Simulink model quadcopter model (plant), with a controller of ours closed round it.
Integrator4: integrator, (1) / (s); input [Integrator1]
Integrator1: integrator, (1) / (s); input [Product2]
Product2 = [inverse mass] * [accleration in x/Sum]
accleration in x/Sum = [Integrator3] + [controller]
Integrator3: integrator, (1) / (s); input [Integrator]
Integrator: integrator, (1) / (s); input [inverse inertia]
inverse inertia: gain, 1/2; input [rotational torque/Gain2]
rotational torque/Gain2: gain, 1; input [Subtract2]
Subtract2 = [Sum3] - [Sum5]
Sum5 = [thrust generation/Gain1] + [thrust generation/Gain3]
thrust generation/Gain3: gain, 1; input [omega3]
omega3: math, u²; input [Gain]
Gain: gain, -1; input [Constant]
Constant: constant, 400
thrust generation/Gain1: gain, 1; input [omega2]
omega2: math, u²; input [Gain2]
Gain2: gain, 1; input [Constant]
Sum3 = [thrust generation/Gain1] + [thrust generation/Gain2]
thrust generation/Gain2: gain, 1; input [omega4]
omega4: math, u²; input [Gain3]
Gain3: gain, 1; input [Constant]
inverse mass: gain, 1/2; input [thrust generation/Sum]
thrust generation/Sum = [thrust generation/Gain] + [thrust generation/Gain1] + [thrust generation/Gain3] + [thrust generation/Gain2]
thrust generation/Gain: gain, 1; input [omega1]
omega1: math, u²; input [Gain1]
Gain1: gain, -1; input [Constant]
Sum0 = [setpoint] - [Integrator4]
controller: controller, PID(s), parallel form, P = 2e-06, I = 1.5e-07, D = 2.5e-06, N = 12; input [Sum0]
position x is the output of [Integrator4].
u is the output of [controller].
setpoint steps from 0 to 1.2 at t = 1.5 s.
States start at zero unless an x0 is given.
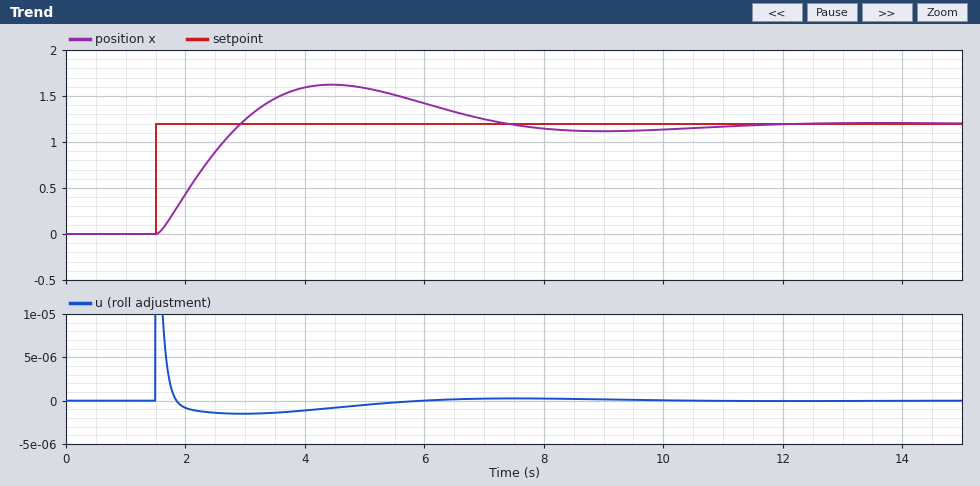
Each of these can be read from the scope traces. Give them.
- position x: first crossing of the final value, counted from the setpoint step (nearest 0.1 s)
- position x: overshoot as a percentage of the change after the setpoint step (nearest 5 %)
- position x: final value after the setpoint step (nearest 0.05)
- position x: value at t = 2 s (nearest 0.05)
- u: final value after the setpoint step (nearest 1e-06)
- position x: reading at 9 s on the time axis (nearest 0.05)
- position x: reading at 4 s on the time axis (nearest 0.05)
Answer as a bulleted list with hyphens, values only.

- 1.4 s
- 35 %
- 1.20
- 0.45
- 0.000000
- 1.10
- 1.60
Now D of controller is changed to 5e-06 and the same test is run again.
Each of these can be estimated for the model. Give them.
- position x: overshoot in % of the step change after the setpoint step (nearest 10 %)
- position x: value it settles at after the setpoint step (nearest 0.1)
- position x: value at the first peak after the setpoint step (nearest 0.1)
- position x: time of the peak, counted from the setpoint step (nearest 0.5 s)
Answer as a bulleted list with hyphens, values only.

- 20 %
- 1.2
- 1.4
- 2.5 s
